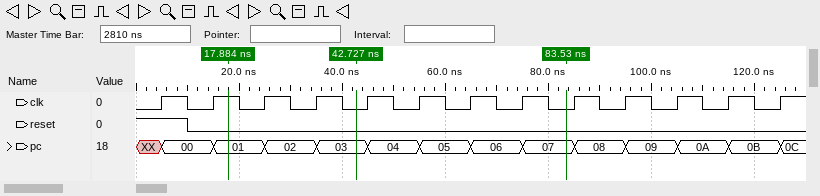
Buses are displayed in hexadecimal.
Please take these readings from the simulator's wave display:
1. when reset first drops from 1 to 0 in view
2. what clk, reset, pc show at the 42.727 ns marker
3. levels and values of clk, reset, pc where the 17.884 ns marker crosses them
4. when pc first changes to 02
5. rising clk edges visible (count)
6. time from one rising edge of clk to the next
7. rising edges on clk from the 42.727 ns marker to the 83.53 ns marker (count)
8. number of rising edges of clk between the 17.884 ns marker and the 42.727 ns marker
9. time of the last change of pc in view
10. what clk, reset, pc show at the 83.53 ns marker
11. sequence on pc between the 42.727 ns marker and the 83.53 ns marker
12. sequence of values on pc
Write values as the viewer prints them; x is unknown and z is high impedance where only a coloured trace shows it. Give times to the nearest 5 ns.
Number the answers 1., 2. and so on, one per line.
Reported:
1. 10 ns
2. clk=0, reset=0, pc=03
3. clk=1, reset=0, pc=01
4. 25 ns
5. 13
6. 10 ns
7. 4
8. 2
9. 125 ns
10. clk=0, reset=0, pc=07
11. 03, 04, 05, 06, 07
12. XX, 00, 01, 02, 03, 04, 05, 06, 07, 08, 09, 0A, 0B, 0C
